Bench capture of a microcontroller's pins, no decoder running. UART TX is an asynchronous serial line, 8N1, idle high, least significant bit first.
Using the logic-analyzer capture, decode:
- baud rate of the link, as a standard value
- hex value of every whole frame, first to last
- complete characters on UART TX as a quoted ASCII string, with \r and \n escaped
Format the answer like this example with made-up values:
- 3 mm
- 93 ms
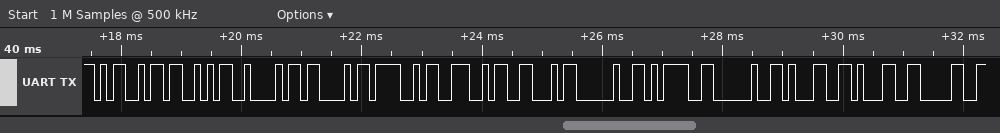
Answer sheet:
- 9600 baud
- 0x4D 0x53 0x42 0x43 0x4F 0x4E 0x46 0x20 0x3D 0x20 0x31 0x31 0x30
- "MSBCONF = 110"
